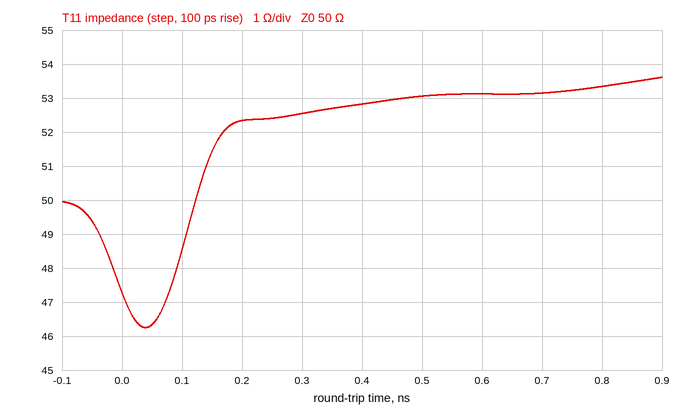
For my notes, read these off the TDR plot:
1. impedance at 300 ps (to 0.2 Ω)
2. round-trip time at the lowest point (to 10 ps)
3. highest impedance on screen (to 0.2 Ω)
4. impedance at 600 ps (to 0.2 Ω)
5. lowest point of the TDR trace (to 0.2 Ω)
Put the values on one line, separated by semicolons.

52.6 Ω; 40 ps; 53.6 Ω; 53.2 Ω; 46.2 Ω
